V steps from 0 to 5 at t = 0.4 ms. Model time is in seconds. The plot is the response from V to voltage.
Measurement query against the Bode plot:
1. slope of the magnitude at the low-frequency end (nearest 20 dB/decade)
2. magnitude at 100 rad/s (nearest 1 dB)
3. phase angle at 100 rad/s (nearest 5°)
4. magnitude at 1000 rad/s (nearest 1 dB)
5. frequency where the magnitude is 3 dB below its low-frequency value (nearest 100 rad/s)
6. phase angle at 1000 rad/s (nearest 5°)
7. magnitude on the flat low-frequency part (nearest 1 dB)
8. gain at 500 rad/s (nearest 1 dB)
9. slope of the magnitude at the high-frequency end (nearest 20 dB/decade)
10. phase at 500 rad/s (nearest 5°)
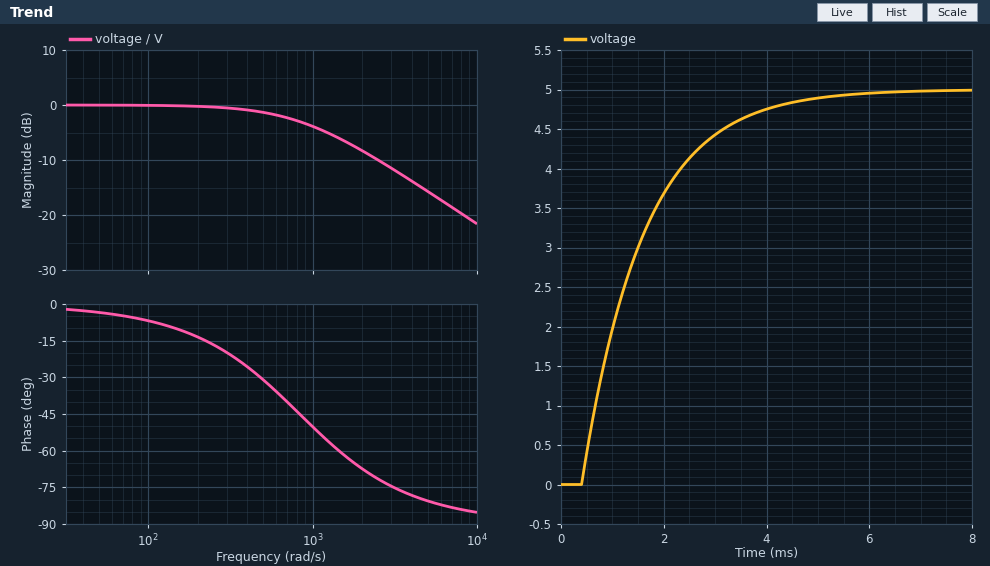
0 dB/decade
0 dB
-5°
-4 dB
800 rad/s
-50°
0 dB
-1 dB
-20 dB/decade
-30°
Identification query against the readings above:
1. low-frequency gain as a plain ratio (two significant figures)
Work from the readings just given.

1.0
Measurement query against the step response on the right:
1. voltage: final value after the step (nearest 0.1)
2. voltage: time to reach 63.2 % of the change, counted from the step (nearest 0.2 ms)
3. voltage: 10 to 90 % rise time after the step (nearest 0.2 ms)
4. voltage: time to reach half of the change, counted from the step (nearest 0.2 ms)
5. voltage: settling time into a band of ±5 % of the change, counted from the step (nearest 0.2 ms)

5.0
1.2 ms
2.6 ms
0.8 ms
3.6 ms
